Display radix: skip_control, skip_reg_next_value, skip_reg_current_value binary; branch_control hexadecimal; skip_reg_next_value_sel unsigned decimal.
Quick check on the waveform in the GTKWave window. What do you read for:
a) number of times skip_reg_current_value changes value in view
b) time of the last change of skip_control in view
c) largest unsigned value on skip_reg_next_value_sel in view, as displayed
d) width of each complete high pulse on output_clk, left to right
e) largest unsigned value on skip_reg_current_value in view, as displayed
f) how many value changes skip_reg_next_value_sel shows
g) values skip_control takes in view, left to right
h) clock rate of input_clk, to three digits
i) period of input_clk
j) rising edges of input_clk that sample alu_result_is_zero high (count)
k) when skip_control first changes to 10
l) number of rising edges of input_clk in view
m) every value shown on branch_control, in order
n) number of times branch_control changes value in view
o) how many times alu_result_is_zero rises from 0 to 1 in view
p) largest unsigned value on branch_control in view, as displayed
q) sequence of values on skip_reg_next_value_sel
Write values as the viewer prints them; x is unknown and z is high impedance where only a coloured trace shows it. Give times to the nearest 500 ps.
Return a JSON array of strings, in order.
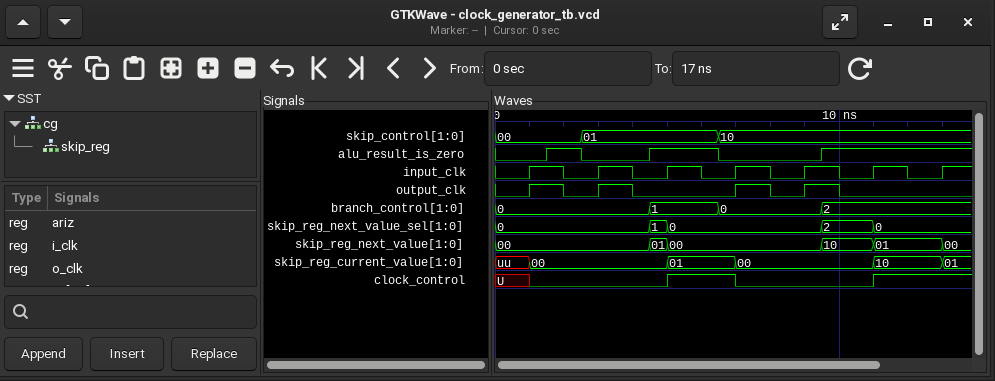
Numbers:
["5", "6500 ps", "2", "1000 ps, 1000 ps, 1000 ps, 1000 ps", "10", "4", "00, 01, 10", "500 MHz", "2000 ps", "3", "6500 ps", "7", "0, 1, 0, 2", "3", "3", "2", "0, 1, 0, 2, 0"]
